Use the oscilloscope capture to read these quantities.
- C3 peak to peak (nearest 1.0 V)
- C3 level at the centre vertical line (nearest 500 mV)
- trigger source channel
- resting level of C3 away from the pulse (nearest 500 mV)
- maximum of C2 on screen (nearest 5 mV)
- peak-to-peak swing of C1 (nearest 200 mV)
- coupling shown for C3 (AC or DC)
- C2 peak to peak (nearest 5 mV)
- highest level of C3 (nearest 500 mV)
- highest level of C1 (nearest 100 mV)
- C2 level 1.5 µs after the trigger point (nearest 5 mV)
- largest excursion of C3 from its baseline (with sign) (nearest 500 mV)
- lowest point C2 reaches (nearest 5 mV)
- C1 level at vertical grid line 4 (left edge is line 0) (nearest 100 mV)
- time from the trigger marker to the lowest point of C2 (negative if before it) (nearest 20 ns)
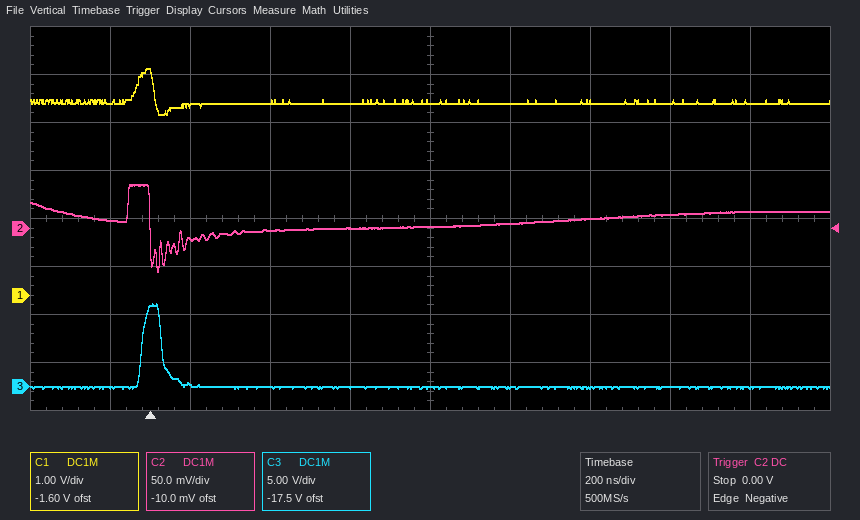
9.0 V
0.0 V
C2
0.0 V
45 mV
1.0 V
DC
90 mV
8.5 V
4.7 V
15 mV
+8.5 V
-45 mV
4.0 V
+20 ns
